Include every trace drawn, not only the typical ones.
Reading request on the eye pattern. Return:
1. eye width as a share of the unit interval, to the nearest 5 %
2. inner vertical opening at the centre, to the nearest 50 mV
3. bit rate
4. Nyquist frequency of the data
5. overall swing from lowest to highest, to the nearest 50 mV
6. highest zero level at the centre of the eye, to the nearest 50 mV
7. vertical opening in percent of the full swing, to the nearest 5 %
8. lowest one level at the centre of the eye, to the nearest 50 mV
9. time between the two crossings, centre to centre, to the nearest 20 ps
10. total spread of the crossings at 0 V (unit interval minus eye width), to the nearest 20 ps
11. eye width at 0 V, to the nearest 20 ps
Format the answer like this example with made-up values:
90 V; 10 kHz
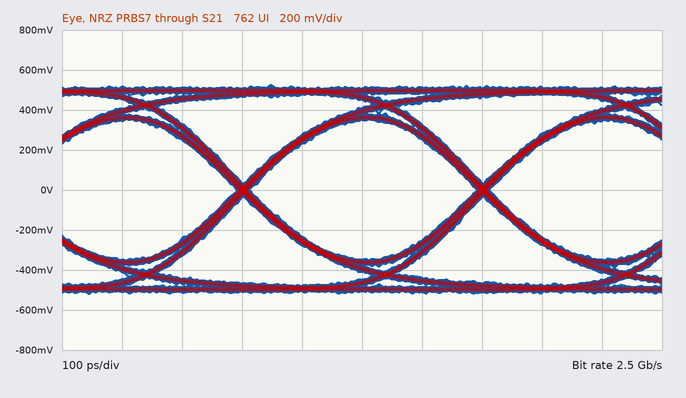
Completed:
95 %; 700 mV; 2.5 Gb/s; 1.25 GHz; 1.05 V; -350 mV; 65 %; 350 mV; 400 ps; 20 ps; 380 ps
